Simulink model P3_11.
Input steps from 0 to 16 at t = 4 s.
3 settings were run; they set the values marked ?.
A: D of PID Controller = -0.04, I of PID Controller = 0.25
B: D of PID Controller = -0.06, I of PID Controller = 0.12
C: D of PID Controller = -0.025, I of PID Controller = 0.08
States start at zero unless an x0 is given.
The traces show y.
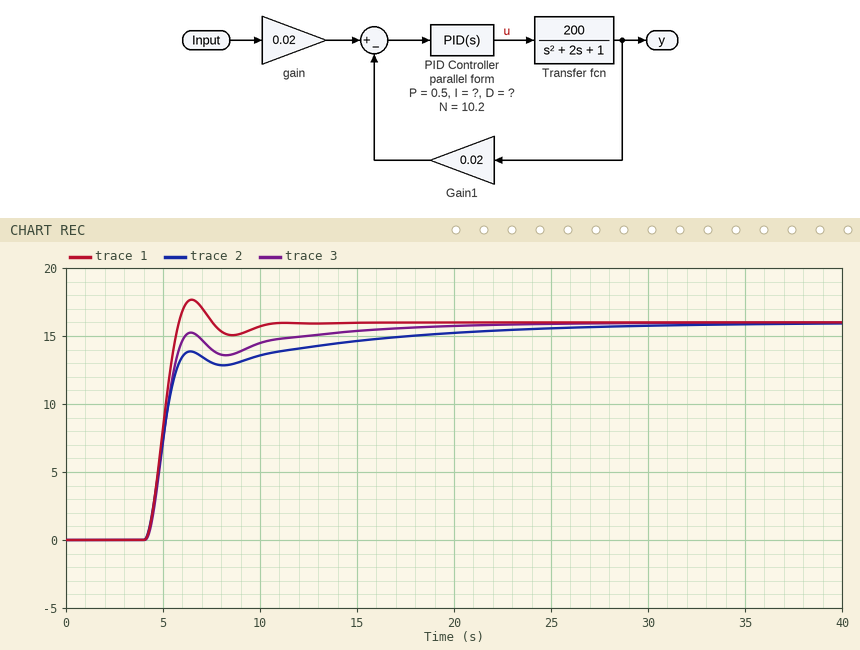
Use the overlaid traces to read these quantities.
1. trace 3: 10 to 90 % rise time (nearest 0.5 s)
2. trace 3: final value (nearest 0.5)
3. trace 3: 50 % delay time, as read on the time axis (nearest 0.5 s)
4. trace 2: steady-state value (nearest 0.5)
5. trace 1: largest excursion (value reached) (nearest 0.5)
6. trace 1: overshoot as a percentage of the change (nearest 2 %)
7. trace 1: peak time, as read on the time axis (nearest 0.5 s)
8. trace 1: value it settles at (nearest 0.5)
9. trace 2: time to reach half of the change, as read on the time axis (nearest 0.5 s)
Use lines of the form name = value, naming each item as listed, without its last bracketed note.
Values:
trace 3: 10 to 90 % rise time = 1.5 s
trace 3: final value = 16.0
trace 3: 50 % delay time, as read on the time axis = 5.0 s
trace 2: steady-state value = 16.0
trace 1: largest excursion (value reached) = 17.5
trace 1: overshoot as a percentage of the change = 10 %
trace 1: peak time, as read on the time axis = 6.5 s
trace 1: value it settles at = 16.0
trace 2: time to reach half of the change, as read on the time axis = 5.0 s
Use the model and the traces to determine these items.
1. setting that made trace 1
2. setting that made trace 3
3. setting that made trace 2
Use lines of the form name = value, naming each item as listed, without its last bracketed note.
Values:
setting that made trace 1 = A
setting that made trace 3 = B
setting that made trace 2 = C
